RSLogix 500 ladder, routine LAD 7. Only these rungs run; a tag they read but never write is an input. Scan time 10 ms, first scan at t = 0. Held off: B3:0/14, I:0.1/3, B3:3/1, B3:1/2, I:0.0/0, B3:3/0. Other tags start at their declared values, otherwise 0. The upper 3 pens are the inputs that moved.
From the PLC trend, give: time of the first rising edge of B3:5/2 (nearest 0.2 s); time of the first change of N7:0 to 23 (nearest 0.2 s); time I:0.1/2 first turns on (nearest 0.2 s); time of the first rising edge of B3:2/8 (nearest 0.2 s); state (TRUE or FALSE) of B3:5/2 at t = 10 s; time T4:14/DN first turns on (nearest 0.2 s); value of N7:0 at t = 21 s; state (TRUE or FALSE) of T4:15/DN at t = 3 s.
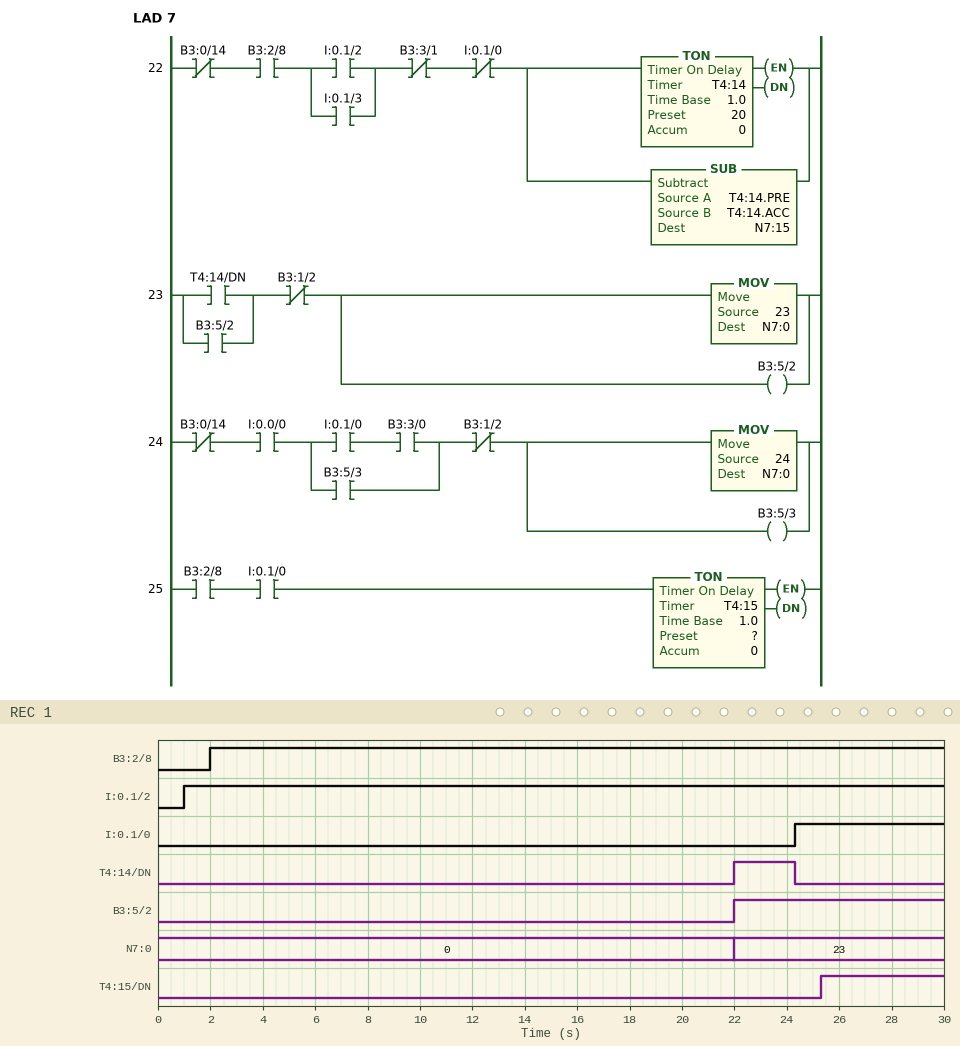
22.0 s
22.0 s
1.0 s
2.0 s
FALSE
22.0 s
0
FALSE
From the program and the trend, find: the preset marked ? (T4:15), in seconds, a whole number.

1 s
